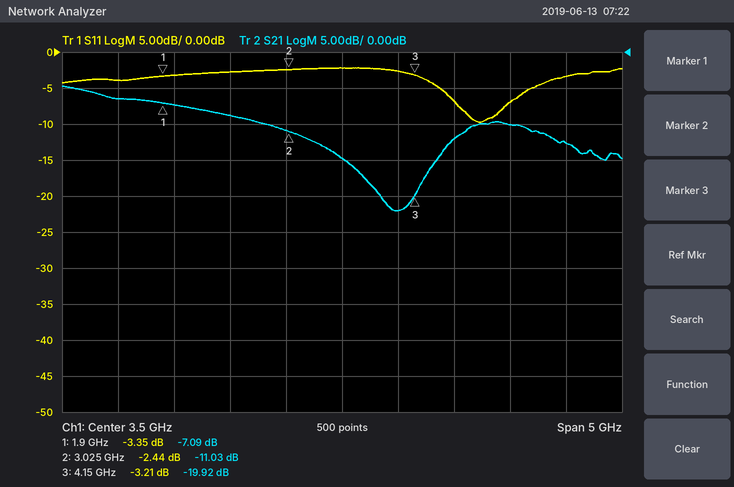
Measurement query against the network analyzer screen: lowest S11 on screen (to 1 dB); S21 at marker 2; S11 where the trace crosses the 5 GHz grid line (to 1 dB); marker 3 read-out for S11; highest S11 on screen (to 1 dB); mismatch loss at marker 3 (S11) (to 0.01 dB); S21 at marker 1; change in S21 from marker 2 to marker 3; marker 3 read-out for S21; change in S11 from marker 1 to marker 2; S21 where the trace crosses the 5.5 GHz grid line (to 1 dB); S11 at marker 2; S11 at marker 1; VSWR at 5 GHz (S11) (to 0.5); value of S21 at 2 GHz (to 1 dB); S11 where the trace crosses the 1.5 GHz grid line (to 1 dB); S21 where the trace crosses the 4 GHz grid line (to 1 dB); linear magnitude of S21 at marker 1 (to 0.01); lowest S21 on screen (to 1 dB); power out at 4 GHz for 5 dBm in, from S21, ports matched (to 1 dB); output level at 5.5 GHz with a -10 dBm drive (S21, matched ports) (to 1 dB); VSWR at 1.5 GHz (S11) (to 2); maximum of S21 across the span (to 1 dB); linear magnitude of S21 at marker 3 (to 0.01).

-10 dB
-11.03 dB
-7 dB
-3.21 dB
-2 dB
2.82 dB
-7.09 dB
-8.89 dB
-19.92 dB
0.91 dB
-13 dB
-2.44 dB
-3.35 dB
2.5
-7 dB
-4 dB
-22 dB
0.44
-22 dB
-17 dBm
-23 dBm
4
-5 dB
0.10
